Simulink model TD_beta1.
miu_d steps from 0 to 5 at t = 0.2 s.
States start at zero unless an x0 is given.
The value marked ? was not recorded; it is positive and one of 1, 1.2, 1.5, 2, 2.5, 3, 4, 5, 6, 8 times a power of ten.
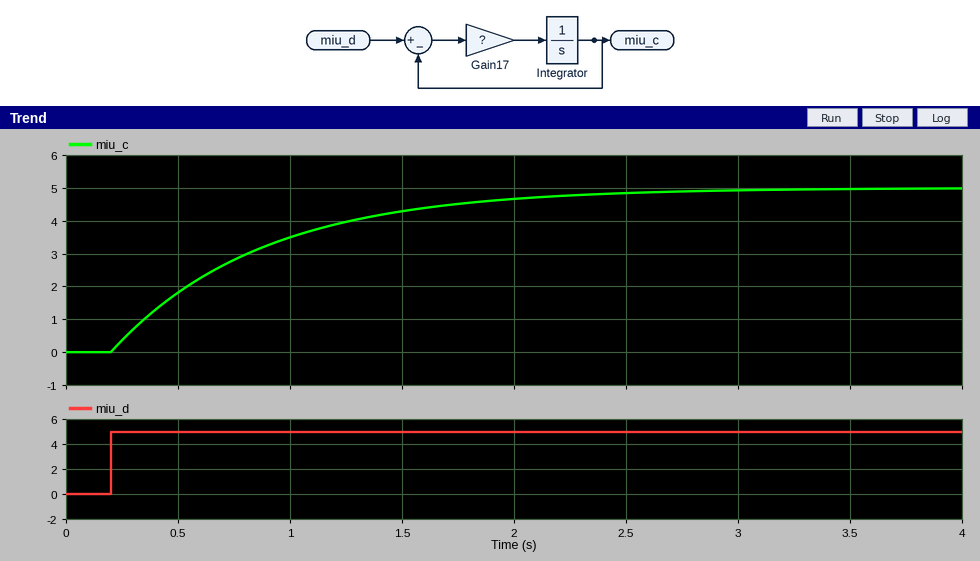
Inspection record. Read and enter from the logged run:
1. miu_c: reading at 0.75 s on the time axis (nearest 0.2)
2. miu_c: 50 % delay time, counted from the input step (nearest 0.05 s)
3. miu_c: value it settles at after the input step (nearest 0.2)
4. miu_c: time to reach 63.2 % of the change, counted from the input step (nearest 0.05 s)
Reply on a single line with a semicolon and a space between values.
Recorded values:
2.8; 0.45 s; 5.0; 0.65 s
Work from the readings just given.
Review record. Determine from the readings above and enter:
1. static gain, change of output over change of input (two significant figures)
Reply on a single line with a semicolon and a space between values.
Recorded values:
1.0
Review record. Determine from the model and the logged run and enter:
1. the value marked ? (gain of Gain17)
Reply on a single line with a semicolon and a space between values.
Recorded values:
1.5
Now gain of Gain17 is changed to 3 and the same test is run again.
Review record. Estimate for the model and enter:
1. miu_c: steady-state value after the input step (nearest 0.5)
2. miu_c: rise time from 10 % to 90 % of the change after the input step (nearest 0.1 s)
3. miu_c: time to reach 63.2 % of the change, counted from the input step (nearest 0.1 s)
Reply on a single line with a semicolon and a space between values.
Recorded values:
5.0; 0.7 s; 0.3 s
